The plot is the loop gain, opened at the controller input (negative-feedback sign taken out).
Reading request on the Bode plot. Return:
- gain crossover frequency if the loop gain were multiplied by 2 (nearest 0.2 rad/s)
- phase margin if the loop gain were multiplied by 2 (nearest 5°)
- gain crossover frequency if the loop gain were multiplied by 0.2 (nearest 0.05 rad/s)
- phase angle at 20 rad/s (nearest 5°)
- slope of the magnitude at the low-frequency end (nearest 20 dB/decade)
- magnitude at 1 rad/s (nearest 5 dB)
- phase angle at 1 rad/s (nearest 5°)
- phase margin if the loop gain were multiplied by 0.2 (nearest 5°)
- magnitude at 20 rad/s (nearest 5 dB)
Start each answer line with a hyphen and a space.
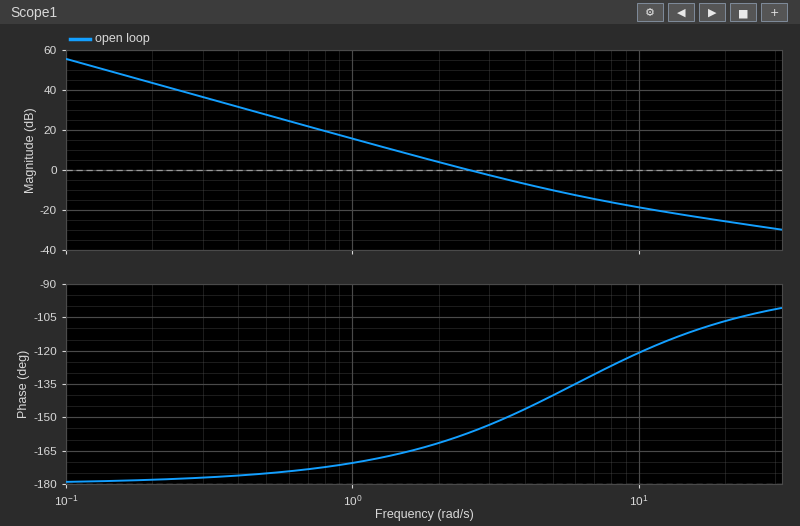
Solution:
- 3.8 rad/s
- 30°
- 1.10 rad/s
- -105°
- -40 dB/decade
- 15 dB
- -170°
- 10°
- -25 dB
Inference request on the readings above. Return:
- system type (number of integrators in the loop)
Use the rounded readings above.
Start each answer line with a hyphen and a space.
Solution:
- 2
